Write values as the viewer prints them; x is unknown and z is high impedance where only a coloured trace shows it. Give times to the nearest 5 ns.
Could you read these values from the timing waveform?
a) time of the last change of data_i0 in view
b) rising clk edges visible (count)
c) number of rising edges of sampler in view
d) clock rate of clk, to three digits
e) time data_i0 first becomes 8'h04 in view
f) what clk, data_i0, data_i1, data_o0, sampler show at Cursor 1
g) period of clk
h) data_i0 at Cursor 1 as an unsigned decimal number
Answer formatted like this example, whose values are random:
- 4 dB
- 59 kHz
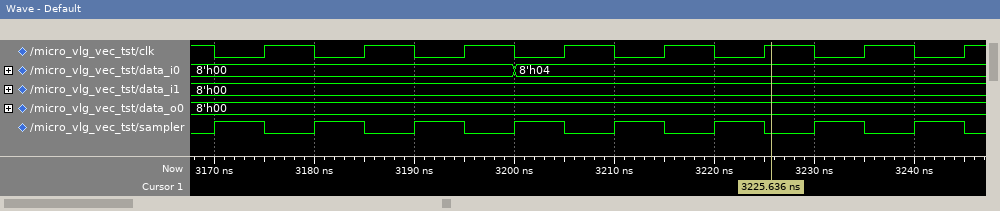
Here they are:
- 3200 ns
- 8
- 8
- 100 MHz
- 3200 ns
- clk=1, data_i0=8'h04, data_i1=8'h00, data_o0=8'h00, sampler=0
- 10 ns
- 4
